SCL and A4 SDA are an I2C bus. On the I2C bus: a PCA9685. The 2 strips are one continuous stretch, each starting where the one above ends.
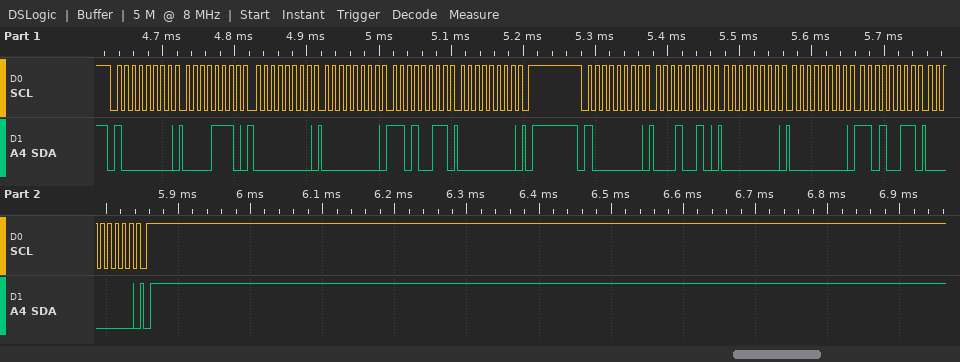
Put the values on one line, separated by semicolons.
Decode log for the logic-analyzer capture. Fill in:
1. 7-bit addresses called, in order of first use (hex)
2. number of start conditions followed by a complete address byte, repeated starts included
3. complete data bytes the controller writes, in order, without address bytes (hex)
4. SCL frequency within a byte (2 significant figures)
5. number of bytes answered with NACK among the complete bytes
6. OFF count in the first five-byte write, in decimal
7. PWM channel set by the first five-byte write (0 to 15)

0x40; 2; 0E 00 00 D3 00 12 00 00 D3 00; 100 kHz; 0; 211; 2
